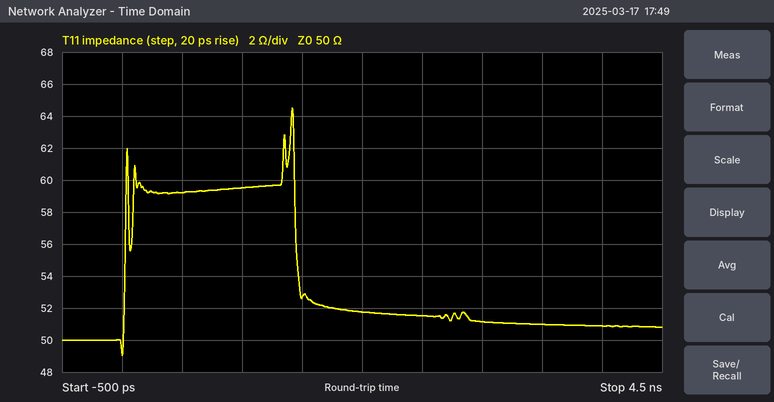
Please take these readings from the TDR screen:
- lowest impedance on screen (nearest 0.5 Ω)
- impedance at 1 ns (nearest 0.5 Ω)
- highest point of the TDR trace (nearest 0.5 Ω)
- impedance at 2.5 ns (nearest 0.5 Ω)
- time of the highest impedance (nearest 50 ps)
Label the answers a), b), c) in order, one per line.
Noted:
a) 49.0 Ω
b) 59.5 Ω
c) 64.5 Ω
d) 51.5 Ω
e) 1.40 ns
